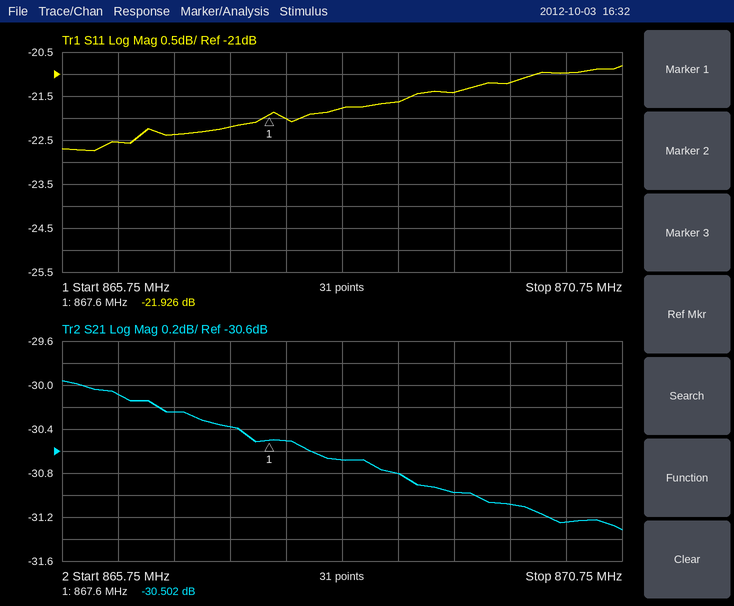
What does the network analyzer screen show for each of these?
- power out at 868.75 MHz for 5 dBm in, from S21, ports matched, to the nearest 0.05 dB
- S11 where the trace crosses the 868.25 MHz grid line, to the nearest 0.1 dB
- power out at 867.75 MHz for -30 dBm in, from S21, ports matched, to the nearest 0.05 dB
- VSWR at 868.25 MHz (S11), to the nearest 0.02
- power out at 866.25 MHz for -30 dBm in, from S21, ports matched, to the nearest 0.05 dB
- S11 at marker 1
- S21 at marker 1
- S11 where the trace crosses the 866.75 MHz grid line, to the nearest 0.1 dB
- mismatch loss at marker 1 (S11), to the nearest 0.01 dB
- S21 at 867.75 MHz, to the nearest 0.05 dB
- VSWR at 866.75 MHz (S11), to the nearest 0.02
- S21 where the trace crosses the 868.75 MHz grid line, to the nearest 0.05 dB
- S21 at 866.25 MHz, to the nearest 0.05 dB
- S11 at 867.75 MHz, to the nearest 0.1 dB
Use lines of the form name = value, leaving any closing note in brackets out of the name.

power out at 868.75 MHz for 5 dBm in, from S21, ports matched, to the nearest 0.05 dB = -25.80 dBm
S11 where the trace crosses the 868.25 MHz grid line, to the nearest 0.1 dB = -21.8 dB
power out at 867.75 MHz for -30 dBm in, from S21, ports matched, to the nearest 0.05 dB = -60.50 dBm
VSWR at 868.25 MHz (S11), to the nearest 0.02 = 1.18
power out at 866.25 MHz for -30 dBm in, from S21, ports matched, to the nearest 0.05 dB = -60.10 dBm
S11 at marker 1 = -21.926 dB
S21 at marker 1 = -30.502 dB
S11 where the trace crosses the 866.75 MHz grid line, to the nearest 0.1 dB = -22.4 dB
mismatch loss at marker 1 (S11), to the nearest 0.01 dB = 0.03 dB
S21 at 867.75 MHz, to the nearest 0.05 dB = -30.50 dB
VSWR at 866.75 MHz (S11), to the nearest 0.02 = 1.16
S21 where the trace crosses the 868.75 MHz grid line, to the nearest 0.05 dB = -30.80 dB
S21 at 866.25 MHz, to the nearest 0.05 dB = -30.10 dB
S11 at 867.75 MHz, to the nearest 0.1 dB = -22.0 dB
